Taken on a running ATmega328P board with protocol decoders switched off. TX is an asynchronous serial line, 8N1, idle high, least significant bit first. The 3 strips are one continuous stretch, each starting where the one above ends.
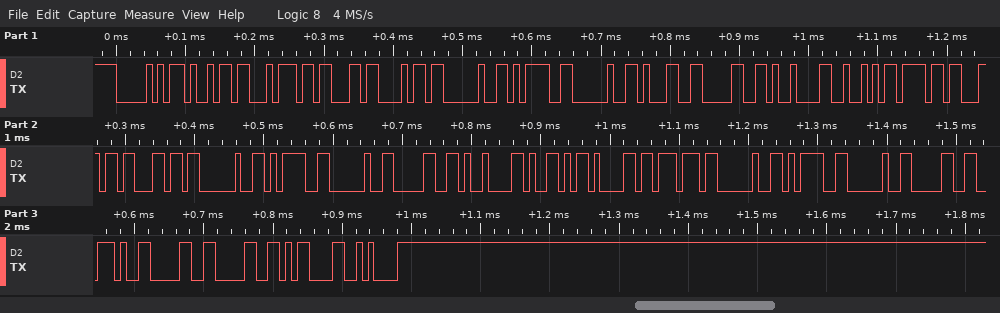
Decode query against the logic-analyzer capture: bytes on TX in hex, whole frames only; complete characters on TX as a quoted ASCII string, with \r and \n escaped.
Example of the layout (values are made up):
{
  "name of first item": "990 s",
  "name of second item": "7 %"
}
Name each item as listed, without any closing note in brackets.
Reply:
{
  "bytes on TX in hex, whole frames only": "0x50 0x69 0x74 0x63 0x68 0x20 0x3D 0x20 0x31 0x30 0x09 0x52 0x6F 0x6C 0x6C 0x20 0x3D 0x20 0x30 0x09 0x59 0x61 0x77 0x20 0x3D 0x20 0x30 0x2E 0x30 0x30 0x0D 0x0A",
  "complete characters on TX as a quoted ASCII string, with \\r and \\n escaped": "\"Pitch = 10\\tRoll = 0\\tYaw = 0.00\\r\\n\""
}
